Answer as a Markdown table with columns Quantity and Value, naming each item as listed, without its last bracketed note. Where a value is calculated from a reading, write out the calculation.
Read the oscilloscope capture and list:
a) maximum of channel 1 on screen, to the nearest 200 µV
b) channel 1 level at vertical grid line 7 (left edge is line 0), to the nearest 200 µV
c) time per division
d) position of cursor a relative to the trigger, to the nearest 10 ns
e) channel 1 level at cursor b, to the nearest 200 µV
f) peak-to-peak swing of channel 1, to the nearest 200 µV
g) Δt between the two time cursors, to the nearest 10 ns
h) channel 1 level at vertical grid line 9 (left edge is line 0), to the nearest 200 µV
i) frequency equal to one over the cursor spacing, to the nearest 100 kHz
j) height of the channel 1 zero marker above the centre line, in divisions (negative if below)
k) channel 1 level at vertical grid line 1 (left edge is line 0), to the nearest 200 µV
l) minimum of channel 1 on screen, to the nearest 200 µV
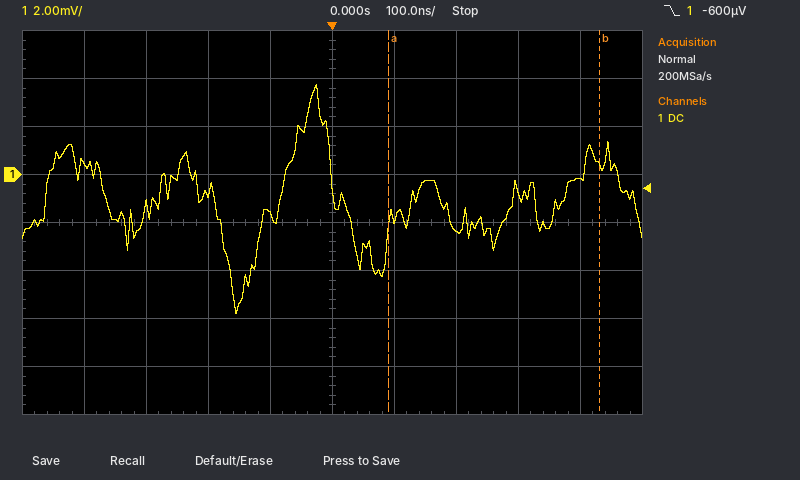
| Quantity | Value |
|---|---|
| maximum of channel 1 on screen, to the nearest 200 µV | 3.8 mV |
| channel 1 level at vertical grid line 7 (left edge is line 0), to the nearest 200 µV | -2.4 mV |
| time per division | 100 ns |
| position of cursor a relative to the trigger, to the nearest 10 ns | +90 ns |
| channel 1 level at cursor b, to the nearest 200 µV | 400 µV |
| peak-to-peak swing of channel 1, to the nearest 200 µV | 3.8 mV − (-5.8 mV) = 9.6 mV |
| Δt between the two time cursors, to the nearest 10 ns | 340 ns |
| channel 1 level at vertical grid line 9 (left edge is line 0), to the nearest 200 µV | -200 µV |
| frequency equal to one over the cursor spacing, to the nearest 100 kHz | 1 / 340 ns ≈ 2.9 MHz |
| height of the channel 1 zero marker above the centre line, in divisions | +1.0 div |
| channel 1 level at vertical grid line 1 (left edge is line 0), to the nearest 200 µV | 400 µV |
| minimum of channel 1 on screen, to the nearest 200 µV | -5.8 mV |
